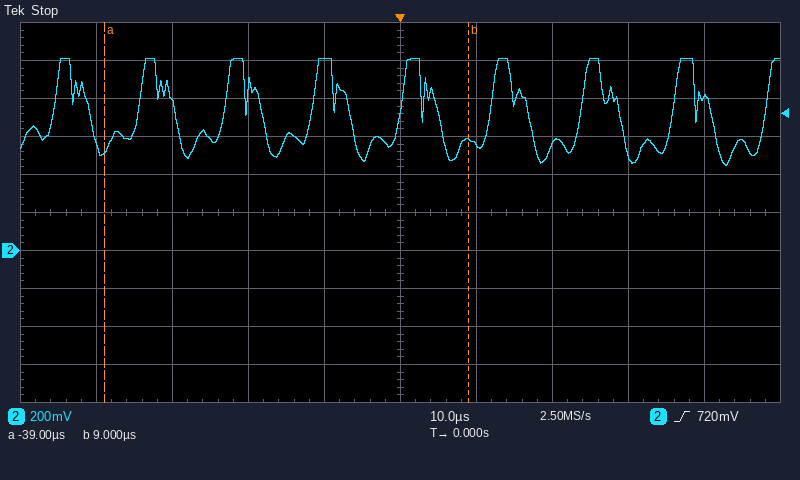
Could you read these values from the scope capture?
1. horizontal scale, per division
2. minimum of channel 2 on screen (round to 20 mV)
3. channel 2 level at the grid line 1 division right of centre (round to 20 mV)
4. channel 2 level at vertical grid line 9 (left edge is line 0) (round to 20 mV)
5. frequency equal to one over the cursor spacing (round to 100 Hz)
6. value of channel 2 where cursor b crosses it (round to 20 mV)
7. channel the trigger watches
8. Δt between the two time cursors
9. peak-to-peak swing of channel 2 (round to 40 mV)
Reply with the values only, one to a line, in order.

10 µs
440 mV
560 mV
800 mV
20.8 kHz
580 mV
channel 2
48 µs
560 mV
